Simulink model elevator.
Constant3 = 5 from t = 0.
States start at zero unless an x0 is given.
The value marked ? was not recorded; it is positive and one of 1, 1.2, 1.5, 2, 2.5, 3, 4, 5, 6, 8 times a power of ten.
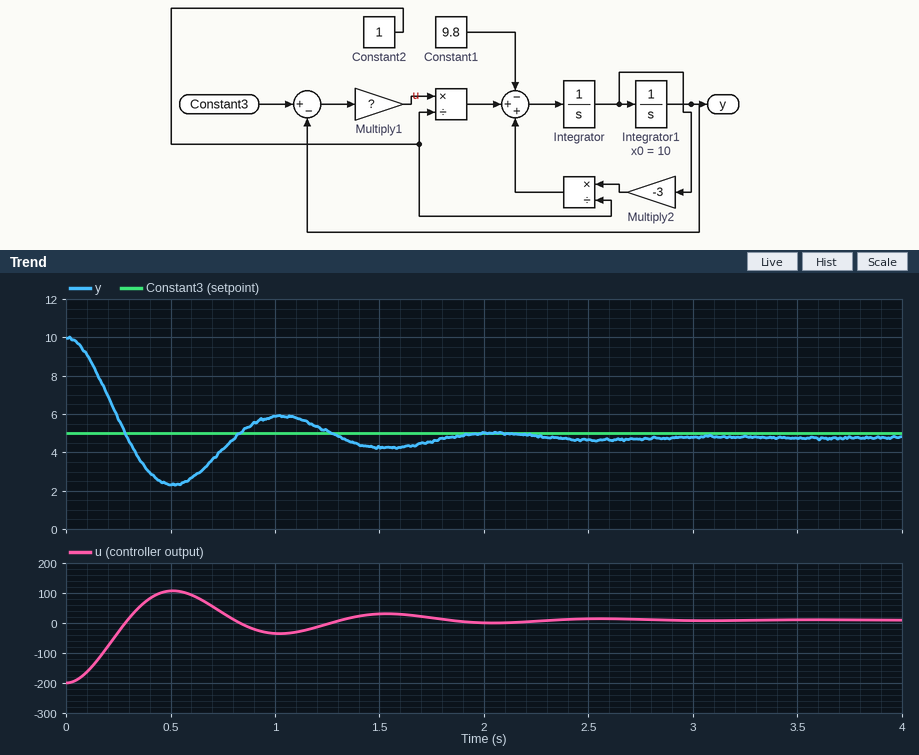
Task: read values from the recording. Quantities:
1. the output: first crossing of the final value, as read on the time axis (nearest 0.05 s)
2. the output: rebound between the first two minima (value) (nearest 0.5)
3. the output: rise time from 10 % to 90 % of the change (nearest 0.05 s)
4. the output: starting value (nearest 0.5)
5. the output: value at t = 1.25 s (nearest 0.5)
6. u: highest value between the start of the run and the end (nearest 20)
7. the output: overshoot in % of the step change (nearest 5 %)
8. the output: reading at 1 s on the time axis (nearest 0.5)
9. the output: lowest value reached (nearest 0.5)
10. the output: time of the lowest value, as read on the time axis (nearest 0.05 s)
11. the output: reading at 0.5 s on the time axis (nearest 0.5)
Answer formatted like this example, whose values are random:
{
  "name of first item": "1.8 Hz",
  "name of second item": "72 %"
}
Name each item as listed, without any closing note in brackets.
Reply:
{
  "the output: first crossing of the final value, as read on the time axis": "0.30 s",
  "the output: rebound between the first two minima (value)": "6.0",
  "the output: rise time from 10 % to 90 % of the change": "0.20 s",
  "the output: starting value": "10.0",
  "the output: value at t = 1.25 s": "5.0",
  "u: highest value between the start of the run and the end": "100",
  "the output: overshoot in % of the step change": "45 %",
  "the output: reading at 1 s on the time axis": "6.0",
  "the output: lowest value reached": "2.5",
  "the output: time of the lowest value, as read on the time axis": "0.50 s",
  "the output: reading at 0.5 s on the time axis": "2.5"
}
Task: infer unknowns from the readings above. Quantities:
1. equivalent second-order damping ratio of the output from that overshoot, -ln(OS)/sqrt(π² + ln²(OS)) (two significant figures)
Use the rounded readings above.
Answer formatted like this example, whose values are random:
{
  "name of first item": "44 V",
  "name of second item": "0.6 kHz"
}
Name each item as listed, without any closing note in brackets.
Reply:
{
  "equivalent second-order damping ratio of the output from that overshoot, -ln(OS)/sqrt(π² + ln²(OS))": "0.25"
}
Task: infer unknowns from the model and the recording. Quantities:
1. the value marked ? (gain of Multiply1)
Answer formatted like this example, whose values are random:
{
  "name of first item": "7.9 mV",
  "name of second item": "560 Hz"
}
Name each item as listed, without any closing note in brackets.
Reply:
{
  "the value marked ?": "40"
}
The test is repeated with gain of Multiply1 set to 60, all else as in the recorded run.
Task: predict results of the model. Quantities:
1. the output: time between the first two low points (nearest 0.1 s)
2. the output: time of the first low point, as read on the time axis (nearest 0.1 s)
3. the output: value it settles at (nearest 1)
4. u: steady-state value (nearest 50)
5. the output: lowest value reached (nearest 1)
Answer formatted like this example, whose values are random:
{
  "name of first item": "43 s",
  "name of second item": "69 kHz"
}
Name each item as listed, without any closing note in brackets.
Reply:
{
  "the output: time between the first two low points": "0.8 s",
  "the output: time of the first low point, as read on the time axis": "0.4 s",
  "the output: value it settles at": "5",
  "u: steady-state value": "0",
  "the output: lowest value reached": "2"
}
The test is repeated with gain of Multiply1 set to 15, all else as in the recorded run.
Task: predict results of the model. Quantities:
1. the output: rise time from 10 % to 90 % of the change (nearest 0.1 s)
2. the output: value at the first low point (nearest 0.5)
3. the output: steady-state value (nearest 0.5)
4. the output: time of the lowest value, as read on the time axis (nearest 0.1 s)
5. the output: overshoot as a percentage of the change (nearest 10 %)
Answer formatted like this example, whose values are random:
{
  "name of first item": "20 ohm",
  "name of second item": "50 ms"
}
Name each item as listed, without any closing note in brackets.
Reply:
{
  "the output: rise time from 10 % to 90 % of the change": "0.4 s",
  "the output: value at the first low point": "3.0",
  "the output: steady-state value": "4.5",
  "the output: time of the lowest value, as read on the time axis": "0.9 s",
  "the output: overshoot as a percentage of the change": "30 %"
}
